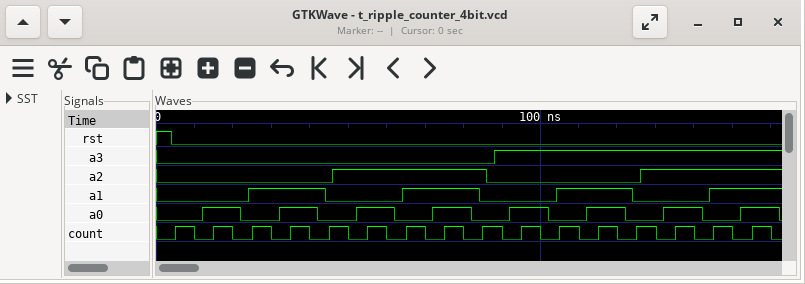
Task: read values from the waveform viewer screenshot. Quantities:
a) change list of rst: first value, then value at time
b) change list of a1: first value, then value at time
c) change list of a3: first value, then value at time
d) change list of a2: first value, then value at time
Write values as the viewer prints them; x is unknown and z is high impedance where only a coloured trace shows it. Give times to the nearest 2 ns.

1, 0 at 4 ns
0, 1 at 24 ns, 0 at 44 ns, 1 at 64 ns, 0 at 84 ns, 1 at 104 ns, 0 at 124 ns, 1 at 144 ns
0, 1 at 88 ns
0, 1 at 46 ns, 0 at 86 ns, 1 at 126 ns
